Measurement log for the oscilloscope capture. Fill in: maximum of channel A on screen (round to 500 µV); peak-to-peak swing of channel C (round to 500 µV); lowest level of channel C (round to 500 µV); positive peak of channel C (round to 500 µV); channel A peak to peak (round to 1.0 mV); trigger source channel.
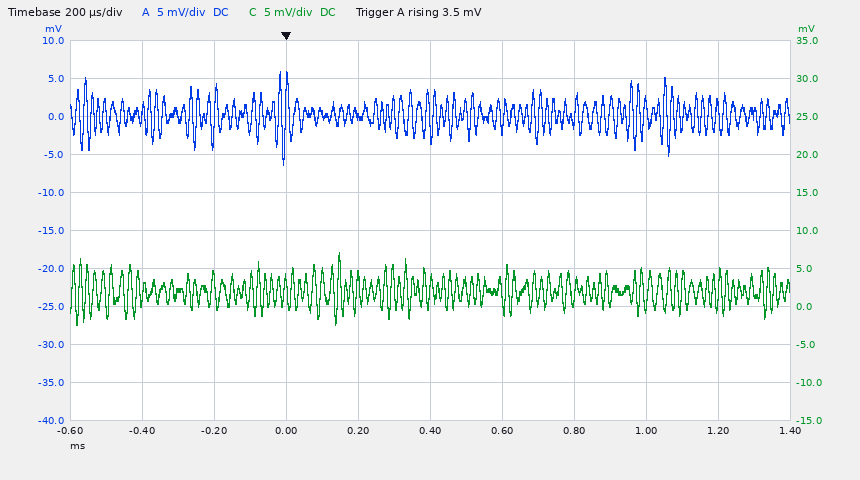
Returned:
6.0 mV
9.5 mV
-2.5 mV
7.0 mV
12.0 mV
channel A
